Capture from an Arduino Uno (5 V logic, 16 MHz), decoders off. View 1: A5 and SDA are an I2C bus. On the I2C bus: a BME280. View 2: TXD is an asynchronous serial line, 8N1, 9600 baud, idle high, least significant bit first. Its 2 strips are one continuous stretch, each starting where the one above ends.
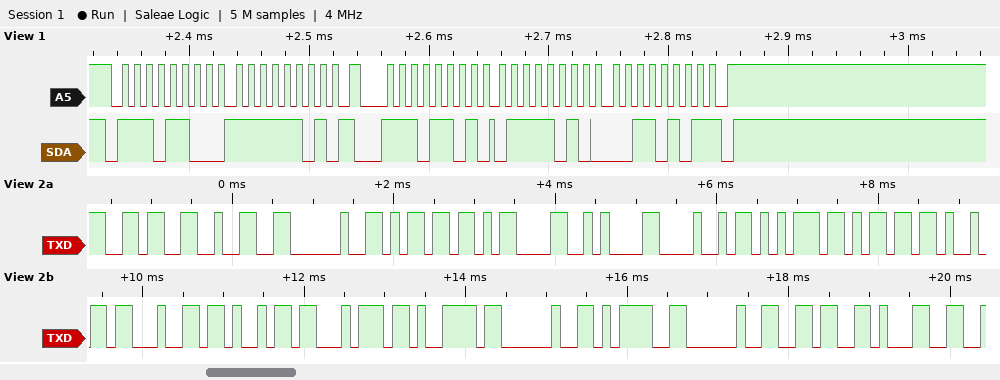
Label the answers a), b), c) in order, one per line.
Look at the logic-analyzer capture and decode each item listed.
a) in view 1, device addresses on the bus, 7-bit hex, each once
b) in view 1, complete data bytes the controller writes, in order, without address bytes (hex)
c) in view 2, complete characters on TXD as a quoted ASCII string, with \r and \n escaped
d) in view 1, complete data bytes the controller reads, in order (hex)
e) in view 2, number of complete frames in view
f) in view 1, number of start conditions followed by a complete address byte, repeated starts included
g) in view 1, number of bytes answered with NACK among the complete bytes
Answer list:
a) 0x76
b) FD
c) "62 m\r\nHumidity = 61"
d) 7A 35
e) 19
f) 2
g) 1
